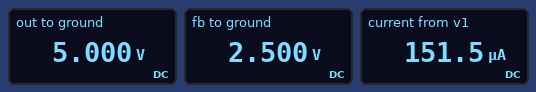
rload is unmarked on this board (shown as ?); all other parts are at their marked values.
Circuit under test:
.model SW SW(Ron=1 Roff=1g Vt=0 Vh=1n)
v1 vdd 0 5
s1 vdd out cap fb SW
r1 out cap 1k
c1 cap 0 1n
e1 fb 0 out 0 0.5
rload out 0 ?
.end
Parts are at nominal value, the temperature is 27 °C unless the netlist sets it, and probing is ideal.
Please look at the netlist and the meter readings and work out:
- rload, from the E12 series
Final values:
33 kΩ
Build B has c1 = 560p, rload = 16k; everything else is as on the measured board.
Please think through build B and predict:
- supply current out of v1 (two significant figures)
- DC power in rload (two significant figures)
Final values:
310 µA
1.6 mW
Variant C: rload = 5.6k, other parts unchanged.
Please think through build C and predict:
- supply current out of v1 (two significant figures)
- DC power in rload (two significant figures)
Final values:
890 µA
4.5 mW
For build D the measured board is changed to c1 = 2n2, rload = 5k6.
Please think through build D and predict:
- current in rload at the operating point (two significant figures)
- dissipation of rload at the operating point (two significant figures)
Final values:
890 µA
4.5 mW
